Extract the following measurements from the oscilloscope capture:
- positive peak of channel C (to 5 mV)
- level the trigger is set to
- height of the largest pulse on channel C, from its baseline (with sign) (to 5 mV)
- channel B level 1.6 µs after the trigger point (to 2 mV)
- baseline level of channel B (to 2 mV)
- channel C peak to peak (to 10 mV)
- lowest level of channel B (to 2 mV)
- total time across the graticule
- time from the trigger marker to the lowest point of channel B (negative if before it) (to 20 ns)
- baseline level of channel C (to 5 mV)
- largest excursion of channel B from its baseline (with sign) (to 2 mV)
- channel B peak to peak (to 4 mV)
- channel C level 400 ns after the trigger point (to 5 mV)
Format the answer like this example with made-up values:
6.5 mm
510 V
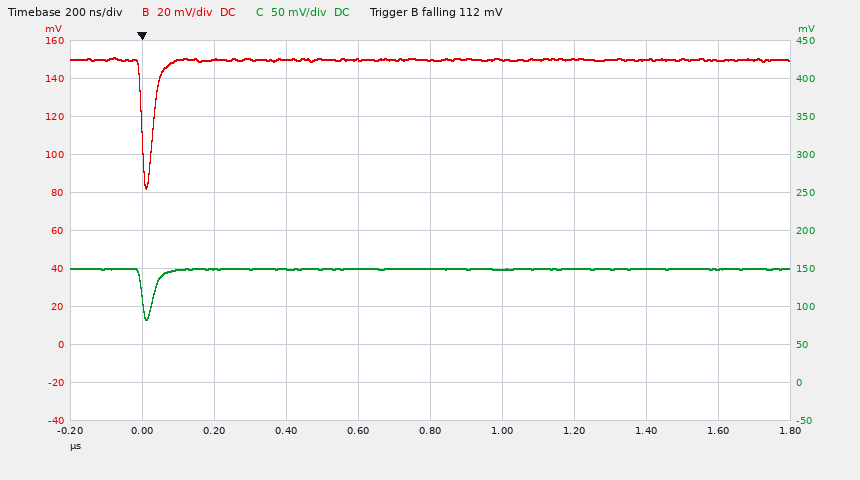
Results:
150 mV
112 mV
-65 mV
150 mV
150 mV
70 mV
82 mV
2 µs
+20 ns
150 mV
-68 mV
68 mV
150 mV
